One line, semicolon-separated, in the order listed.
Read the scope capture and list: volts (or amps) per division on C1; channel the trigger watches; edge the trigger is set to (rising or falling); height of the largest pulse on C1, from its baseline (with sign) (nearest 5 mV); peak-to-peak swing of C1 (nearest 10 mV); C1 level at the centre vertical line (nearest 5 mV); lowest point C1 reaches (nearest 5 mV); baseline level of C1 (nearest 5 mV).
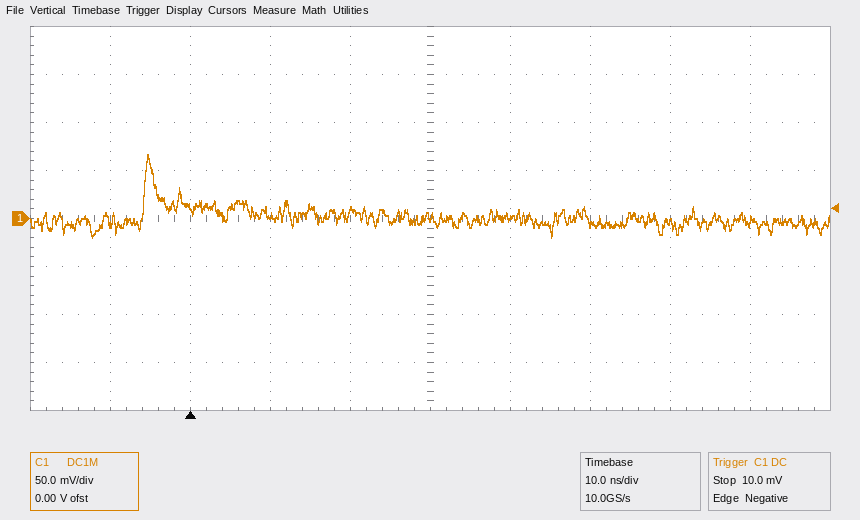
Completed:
50 mV; C1; falling; +70 mV; 90 mV; 0 mV; -20 mV; 0 mV
